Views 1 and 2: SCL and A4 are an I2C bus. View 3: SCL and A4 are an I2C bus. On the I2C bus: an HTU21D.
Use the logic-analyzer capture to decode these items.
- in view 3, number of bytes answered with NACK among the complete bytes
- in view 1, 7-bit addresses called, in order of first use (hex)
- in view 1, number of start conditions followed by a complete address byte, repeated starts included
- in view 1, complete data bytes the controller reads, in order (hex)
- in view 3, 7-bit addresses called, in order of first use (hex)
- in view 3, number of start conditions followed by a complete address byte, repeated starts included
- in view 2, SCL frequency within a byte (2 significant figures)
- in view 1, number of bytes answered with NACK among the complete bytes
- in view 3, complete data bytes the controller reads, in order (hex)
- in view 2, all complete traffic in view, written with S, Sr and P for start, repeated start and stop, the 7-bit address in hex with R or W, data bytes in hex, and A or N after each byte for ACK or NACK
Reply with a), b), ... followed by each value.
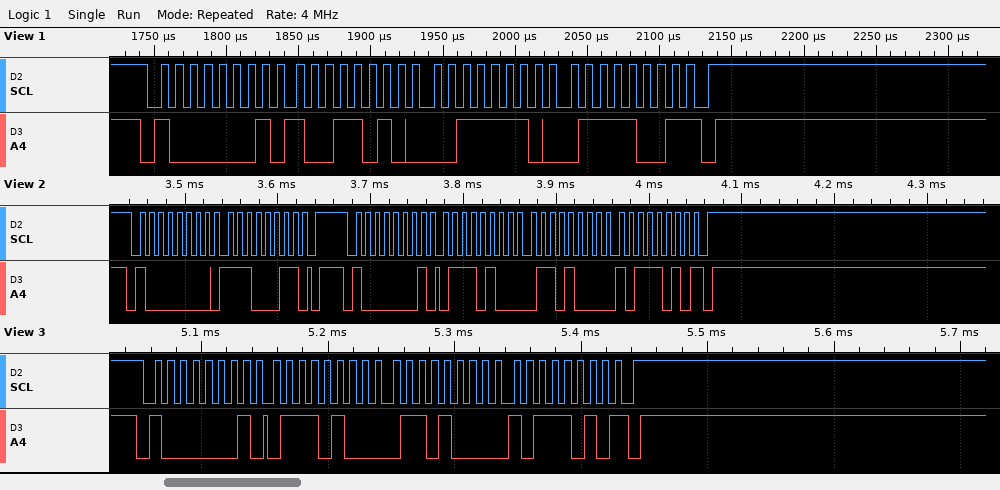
a) 1
b) 0x40
c) 1
d) 9A 3E 79
e) 0x40
f) 1
g) 100 kHz
h) 1
i) 74 68 BA
j) S 40W A E3 A P S 40R A 74 A 68 A BA N P
